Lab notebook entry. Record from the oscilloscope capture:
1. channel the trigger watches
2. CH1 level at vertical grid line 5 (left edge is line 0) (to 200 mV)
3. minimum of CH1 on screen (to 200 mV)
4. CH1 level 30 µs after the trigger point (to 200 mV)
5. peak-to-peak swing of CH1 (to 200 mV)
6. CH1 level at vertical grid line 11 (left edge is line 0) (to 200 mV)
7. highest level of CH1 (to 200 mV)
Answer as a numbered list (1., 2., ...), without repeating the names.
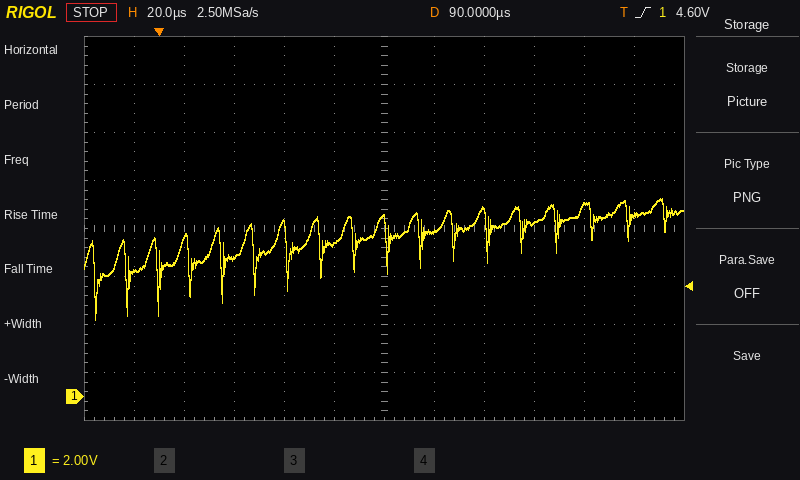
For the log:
1. CH1
2. 6.4 V
3. 3.2 V
4. 5.8 V
5. 5.0 V
6. 7.6 V
7. 8.2 V
